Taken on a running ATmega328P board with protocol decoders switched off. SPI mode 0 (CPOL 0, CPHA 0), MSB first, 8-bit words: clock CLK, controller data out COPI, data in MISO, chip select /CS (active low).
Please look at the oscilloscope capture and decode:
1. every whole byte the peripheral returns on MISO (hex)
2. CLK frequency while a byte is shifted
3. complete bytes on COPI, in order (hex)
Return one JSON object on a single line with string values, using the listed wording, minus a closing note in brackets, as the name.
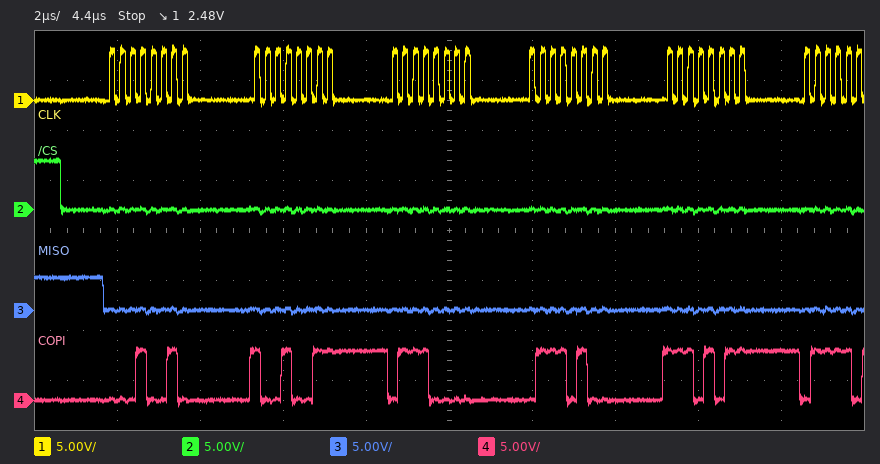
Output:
{"every whole byte the peripheral returns on MISO": "00 00 00 00 00", "CLK frequency while a byte is shifted": "4 MHz", "complete bytes on COPI, in order": "12 93 70 74 EB"}
